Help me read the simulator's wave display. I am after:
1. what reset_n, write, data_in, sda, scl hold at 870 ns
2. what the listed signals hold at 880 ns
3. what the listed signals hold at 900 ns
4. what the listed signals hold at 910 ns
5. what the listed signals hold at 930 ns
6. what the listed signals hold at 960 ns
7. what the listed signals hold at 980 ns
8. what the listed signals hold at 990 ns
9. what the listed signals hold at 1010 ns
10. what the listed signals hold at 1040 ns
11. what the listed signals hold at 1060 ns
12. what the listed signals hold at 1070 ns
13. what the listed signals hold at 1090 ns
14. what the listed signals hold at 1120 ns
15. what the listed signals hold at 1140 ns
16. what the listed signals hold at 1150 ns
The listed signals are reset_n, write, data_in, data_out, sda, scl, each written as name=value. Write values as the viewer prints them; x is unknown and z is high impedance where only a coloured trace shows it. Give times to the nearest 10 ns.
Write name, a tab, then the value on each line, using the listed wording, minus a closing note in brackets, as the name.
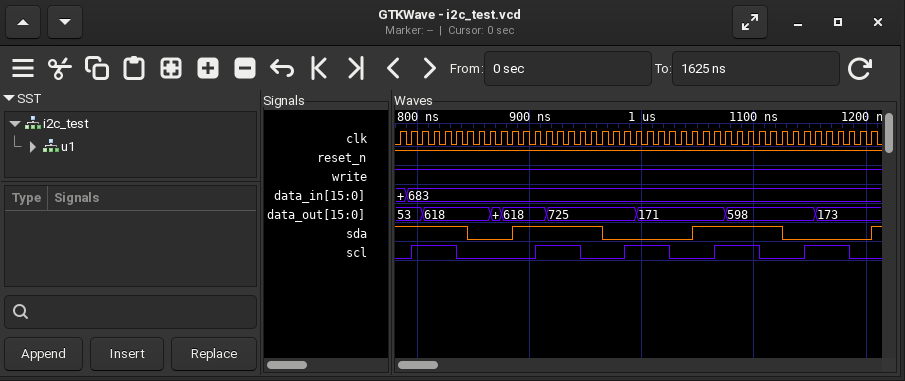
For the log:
what reset_n, write, data_in, sda, scl hold at 870 ns	reset_n=1, write=1, data_in=683, sda=0, scl=0
what the listed signals hold at 880 ns	reset_n=1, write=1, data_in=683, data_out=618, sda=0, scl=0
what the listed signals hold at 900 ns	reset_n=1, write=1, data_in=683, data_out=618, sda=1, scl=0
what the listed signals hold at 910 ns	reset_n=1, write=1, data_in=683, data_out=618, sda=1, scl=1
what the listed signals hold at 930 ns	reset_n=1, write=1, data_in=683, data_out=725, sda=1, scl=1
what the listed signals hold at 960 ns	reset_n=1, write=1, data_in=683, data_out=725, sda=1, scl=0
what the listed signals hold at 980 ns	reset_n=1, write=1, data_in=683, data_out=725, sda=0, scl=0
what the listed signals hold at 990 ns	reset_n=1, write=1, data_in=683, data_out=725, sda=0, scl=1
what the listed signals hold at 1010 ns	reset_n=1, write=1, data_in=683, data_out=171, sda=0, scl=1
what the listed signals hold at 1040 ns	reset_n=1, write=1, data_in=683, data_out=171, sda=0, scl=0
what the listed signals hold at 1060 ns	reset_n=1, write=1, data_in=683, data_out=171, sda=1, scl=0
what the listed signals hold at 1070 ns	reset_n=1, write=1, data_in=683, data_out=171, sda=1, scl=1
what the listed signals hold at 1090 ns	reset_n=1, write=1, data_in=683, data_out=598, sda=1, scl=1
what the listed signals hold at 1120 ns	reset_n=1, write=1, data_in=683, data_out=598, sda=1, scl=0
what the listed signals hold at 1140 ns	reset_n=1, write=1, data_in=683, data_out=598, sda=0, scl=0
what the listed signals hold at 1150 ns	reset_n=1, write=1, data_in=683, data_out=598, sda=0, scl=1
